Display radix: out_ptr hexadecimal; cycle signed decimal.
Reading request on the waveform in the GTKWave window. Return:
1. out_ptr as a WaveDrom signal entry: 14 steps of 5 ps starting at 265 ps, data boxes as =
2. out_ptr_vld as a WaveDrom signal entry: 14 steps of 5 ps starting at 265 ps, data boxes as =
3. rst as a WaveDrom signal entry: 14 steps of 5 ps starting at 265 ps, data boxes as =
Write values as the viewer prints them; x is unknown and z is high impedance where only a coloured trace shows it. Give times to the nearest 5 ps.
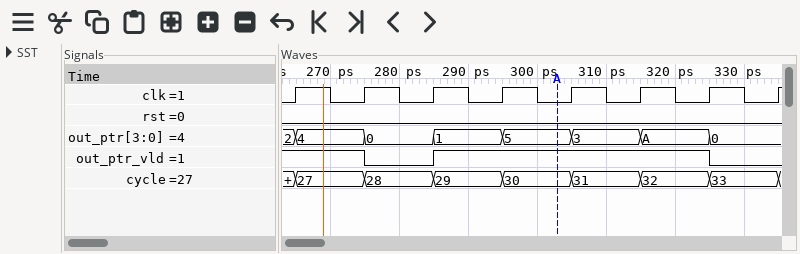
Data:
{name: 'out_ptr', wave: '=.=.=.=.=.=.=.', data: '4 0 1 5 3 A 0'}
{name: 'out_ptr_vld', wave: '1.0.1.......0.'}
{name: 'rst', wave: '0.............'}
